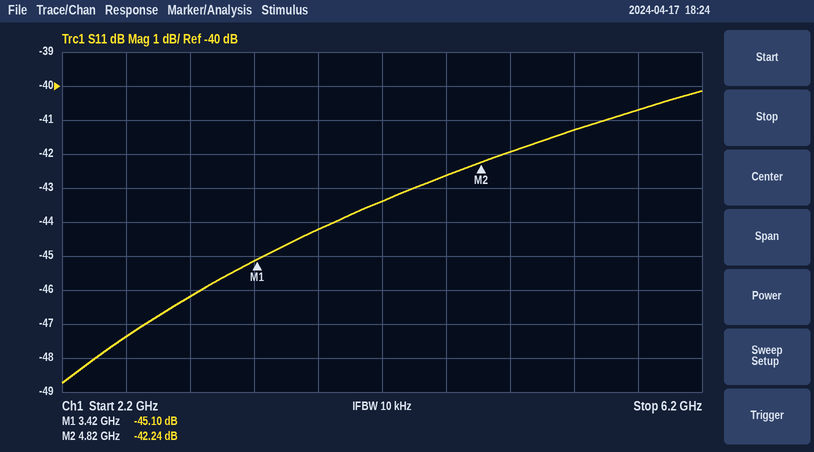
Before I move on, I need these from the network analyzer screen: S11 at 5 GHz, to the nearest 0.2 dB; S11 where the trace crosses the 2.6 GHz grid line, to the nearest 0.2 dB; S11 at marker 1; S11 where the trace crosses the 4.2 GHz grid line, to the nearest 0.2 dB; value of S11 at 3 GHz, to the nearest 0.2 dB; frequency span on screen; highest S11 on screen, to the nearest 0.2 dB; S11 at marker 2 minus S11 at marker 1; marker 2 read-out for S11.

-42.0 dB
-47.4 dB
-45.10 dB
-43.4 dB
-46.2 dB
4 GHz
-40.2 dB
2.86 dB
-42.24 dB
